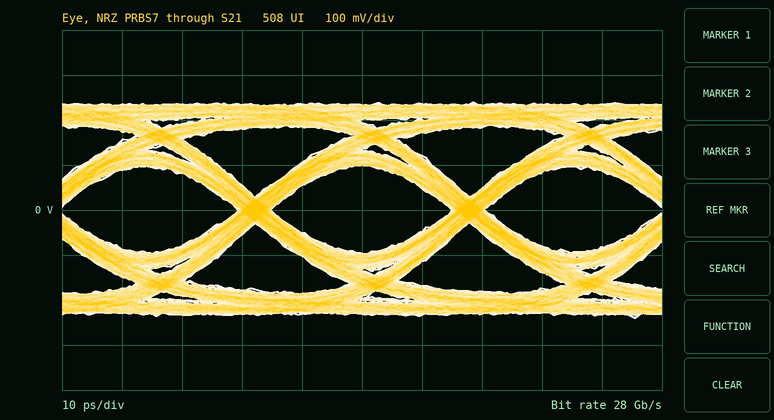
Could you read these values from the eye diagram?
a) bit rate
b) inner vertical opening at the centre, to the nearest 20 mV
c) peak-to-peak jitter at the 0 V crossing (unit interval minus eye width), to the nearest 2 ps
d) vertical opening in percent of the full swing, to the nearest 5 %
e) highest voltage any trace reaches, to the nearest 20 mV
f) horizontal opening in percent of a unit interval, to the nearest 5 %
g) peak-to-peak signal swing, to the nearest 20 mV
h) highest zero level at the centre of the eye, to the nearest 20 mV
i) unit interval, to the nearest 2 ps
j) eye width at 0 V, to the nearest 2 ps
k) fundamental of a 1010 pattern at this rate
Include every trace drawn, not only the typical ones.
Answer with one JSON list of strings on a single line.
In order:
["28 Gb/s", "200 mV", "6 ps", "40 %", "240 mV", "85 %", "480 mV", "-100 mV", "36 ps", "30 ps", "14 GHz"]
